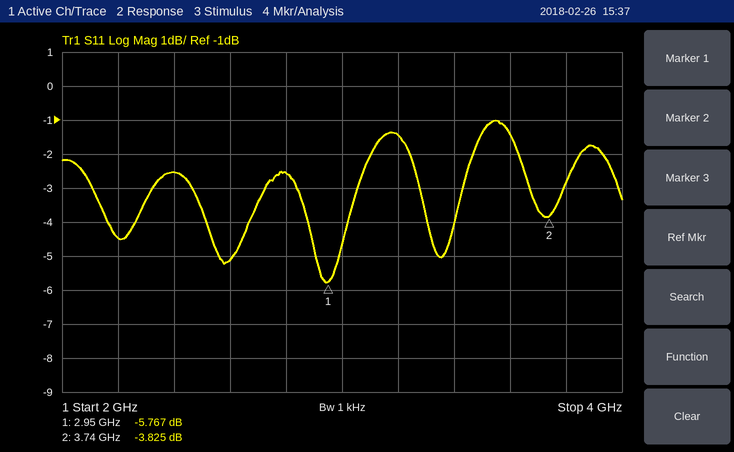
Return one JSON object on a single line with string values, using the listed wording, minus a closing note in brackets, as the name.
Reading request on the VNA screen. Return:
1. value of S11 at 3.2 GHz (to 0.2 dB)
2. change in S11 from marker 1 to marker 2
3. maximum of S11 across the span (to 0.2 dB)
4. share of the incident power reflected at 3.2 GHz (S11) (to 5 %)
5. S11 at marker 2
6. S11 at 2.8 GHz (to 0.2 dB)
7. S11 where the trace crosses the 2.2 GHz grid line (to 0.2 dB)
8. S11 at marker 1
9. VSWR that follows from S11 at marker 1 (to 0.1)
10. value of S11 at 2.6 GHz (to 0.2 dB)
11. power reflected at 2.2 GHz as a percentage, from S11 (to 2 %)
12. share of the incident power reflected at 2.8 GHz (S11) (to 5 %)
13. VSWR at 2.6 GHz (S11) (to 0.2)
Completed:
{"value of S11 at 3.2 GHz": "-1.4 dB", "change in S11 from marker 1 to marker 2": "1.942 dB", "maximum of S11 across the span": "-1.0 dB", "share of the incident power reflected at 3.2 GHz (S11)": "70 %", "S11 at marker 2": "-3.825 dB", "S11 at 2.8 GHz": "-2.6 dB", "S11 where the trace crosses the 2.2 GHz grid line": "-4.4 dB", "S11 at marker 1": "-5.767 dB", "VSWR that follows from S11 at marker 1": "3.1", "value of S11 at 2.6 GHz": "-5.2 dB", "power reflected at 2.2 GHz as a percentage, from S11": "36 %", "share of the incident power reflected at 2.8 GHz (S11)": "55 %", "VSWR at 2.6 GHz (S11)": "3.4"}
